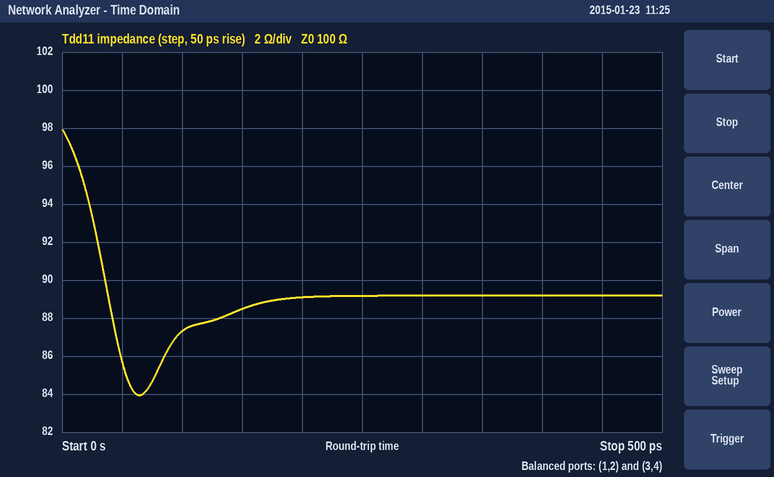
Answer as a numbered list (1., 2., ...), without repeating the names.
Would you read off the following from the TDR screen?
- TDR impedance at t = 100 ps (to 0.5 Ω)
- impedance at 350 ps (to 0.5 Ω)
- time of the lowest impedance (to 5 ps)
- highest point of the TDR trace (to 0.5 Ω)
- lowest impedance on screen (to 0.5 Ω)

1. 87.5 Ω
2. 89.0 Ω
3. 65 ps
4. 98.0 Ω
5. 84.0 Ω
